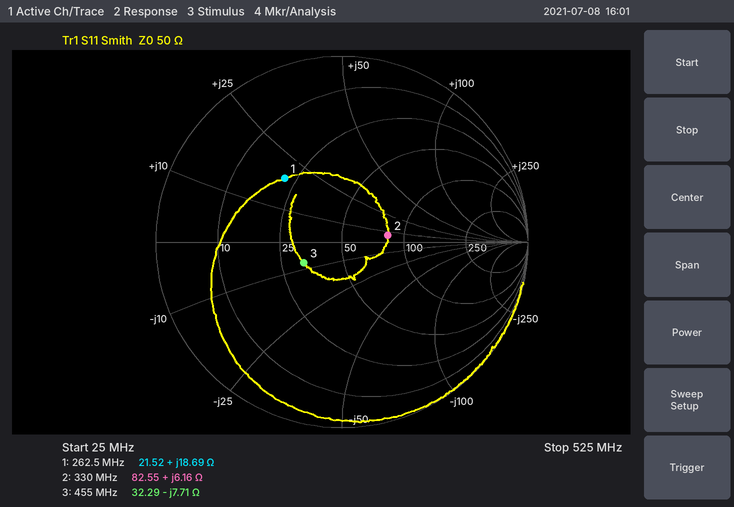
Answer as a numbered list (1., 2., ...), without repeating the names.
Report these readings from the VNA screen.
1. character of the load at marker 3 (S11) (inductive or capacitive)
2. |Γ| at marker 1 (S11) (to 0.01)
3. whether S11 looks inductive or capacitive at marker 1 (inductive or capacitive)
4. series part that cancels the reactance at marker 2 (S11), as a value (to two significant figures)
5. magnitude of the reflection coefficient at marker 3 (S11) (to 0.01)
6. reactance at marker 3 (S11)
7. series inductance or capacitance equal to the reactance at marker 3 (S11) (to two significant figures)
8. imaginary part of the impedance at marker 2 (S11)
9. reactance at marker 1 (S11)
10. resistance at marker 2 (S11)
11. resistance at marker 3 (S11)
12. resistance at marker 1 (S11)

1. capacitive
2. 0.46
3. inductive
4. 78 pF
5. 0.23
6. -7.71 Ω
7. 45 pF
8. +6.16 Ω
9. +18.69 Ω
10. 82.55 Ω
11. 32.29 Ω
12. 21.52 Ω
